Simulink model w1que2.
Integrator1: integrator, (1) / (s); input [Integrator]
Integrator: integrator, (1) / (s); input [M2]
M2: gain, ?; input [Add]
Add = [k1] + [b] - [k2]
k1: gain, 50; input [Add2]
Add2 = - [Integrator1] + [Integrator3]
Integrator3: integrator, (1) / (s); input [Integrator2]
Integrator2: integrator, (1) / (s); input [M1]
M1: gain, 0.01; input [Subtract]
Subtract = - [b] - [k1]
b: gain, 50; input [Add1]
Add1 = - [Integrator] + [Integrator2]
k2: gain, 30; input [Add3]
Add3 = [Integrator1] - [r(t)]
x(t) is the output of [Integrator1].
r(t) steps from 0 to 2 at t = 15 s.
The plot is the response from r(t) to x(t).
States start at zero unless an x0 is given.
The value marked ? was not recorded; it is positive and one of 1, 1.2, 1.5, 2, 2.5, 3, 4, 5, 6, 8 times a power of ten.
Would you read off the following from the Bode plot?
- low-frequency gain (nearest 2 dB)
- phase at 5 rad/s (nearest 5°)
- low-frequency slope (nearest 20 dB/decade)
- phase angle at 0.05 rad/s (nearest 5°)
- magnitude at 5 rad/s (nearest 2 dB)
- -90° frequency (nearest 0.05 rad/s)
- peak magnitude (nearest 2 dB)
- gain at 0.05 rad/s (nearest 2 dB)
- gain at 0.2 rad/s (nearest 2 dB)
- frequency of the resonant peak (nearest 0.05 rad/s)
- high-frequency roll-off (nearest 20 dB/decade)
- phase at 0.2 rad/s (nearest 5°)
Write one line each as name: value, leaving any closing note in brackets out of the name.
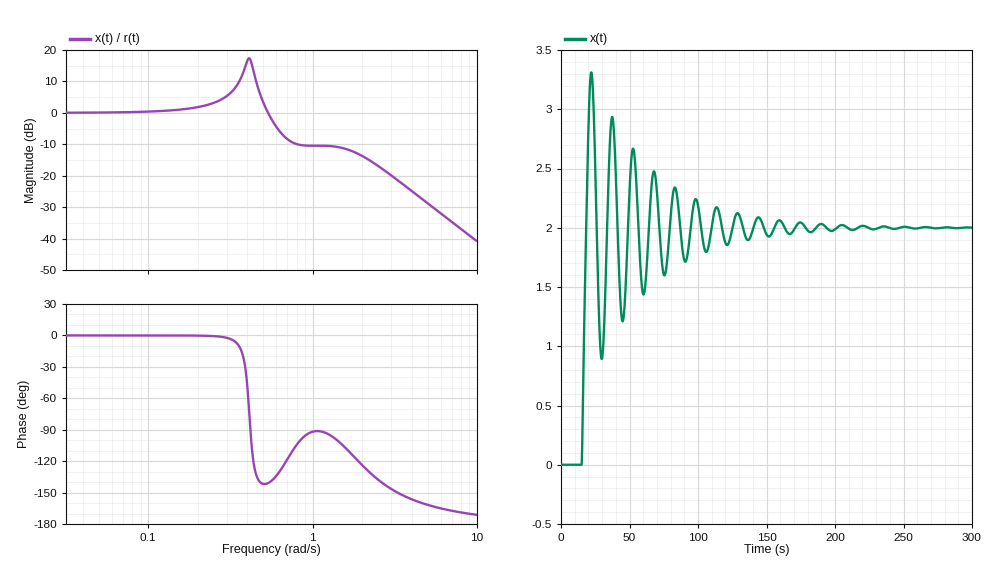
low-frequency gain: 0 dB
phase at 5 rad/s: -160°
low-frequency slope: 0 dB/decade
phase angle at 0.05 rad/s: 0°
magnitude at 5 rad/s: -28 dB
-90° frequency: 0.40 rad/s
peak magnitude: 18 dB
gain at 0.05 rad/s: 0 dB
gain at 0.2 rad/s: 2 dB
frequency of the resonant peak: 0.40 rad/s
high-frequency roll-off: -40 dB/decade
phase at 0.2 rad/s: 0°
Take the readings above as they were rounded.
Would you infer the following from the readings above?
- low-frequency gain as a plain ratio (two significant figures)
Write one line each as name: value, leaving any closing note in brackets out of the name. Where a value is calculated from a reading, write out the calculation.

low-frequency gain as a plain ratio: 10^(0 / 20) = 1.0
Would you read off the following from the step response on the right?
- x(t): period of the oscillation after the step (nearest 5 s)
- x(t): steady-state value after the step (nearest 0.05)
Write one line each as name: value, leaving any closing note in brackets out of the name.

x(t): period of the oscillation after the step: 15 s
x(t): steady-state value after the step: 2.00
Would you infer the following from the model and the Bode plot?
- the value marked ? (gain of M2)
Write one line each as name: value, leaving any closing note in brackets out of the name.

the value marked ?: 0.03
